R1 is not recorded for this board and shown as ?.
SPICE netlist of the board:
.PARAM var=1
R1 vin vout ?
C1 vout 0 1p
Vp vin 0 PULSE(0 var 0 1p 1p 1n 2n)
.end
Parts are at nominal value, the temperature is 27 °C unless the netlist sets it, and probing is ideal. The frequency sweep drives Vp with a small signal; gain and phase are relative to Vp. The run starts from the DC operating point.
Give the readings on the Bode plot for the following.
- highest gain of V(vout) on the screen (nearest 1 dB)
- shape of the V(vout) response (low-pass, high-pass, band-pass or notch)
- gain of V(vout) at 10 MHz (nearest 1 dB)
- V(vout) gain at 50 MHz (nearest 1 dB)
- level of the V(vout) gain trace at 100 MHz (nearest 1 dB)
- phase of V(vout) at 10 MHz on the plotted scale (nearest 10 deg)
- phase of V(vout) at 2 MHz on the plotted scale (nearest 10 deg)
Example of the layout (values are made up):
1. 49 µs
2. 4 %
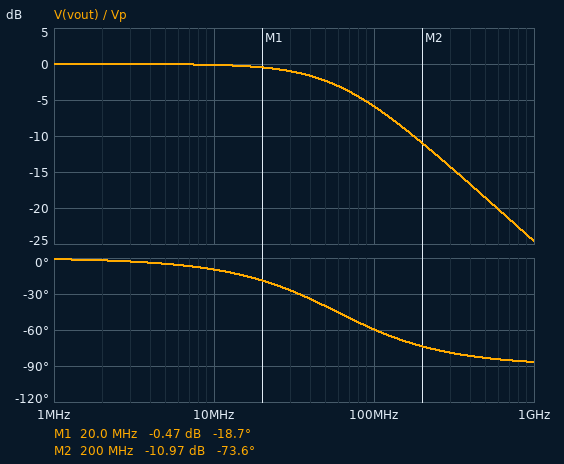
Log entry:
1. 0 dB
2. low-pass
3. 0 dB
4. -2 dB
5. -6 dB
6. -10 deg
7. 0 deg
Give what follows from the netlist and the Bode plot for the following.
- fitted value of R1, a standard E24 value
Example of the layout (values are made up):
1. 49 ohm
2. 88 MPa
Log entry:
1. 2.7 kΩ
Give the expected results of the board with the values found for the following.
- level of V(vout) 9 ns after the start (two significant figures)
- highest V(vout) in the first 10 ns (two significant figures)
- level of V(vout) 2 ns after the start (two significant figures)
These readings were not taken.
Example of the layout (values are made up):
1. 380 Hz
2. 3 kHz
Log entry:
1. 580 mV
2. 580 mV
3. 210 mV
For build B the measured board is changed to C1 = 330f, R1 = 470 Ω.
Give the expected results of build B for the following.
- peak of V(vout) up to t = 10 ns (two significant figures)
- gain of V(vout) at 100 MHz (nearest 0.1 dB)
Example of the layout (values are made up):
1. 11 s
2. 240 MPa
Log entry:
1. 1.0 V
2. 0 dB
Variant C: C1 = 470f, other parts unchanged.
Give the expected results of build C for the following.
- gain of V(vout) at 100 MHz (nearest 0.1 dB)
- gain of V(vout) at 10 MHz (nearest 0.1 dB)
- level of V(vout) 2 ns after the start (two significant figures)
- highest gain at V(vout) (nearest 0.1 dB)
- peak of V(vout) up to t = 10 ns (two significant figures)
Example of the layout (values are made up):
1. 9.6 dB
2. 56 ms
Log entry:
1. -2.1 dB
2. 0 dB
3. 250 mV
4. 0 dB
5. 690 mV
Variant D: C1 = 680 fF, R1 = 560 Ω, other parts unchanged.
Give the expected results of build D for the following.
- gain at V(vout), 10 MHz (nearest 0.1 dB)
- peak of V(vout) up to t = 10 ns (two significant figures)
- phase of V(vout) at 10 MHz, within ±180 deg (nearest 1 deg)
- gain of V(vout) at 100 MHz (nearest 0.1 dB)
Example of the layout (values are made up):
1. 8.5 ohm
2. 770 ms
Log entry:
1. 0 dB
2. 930 mV
3. -1 deg
4. -0.2 dB
